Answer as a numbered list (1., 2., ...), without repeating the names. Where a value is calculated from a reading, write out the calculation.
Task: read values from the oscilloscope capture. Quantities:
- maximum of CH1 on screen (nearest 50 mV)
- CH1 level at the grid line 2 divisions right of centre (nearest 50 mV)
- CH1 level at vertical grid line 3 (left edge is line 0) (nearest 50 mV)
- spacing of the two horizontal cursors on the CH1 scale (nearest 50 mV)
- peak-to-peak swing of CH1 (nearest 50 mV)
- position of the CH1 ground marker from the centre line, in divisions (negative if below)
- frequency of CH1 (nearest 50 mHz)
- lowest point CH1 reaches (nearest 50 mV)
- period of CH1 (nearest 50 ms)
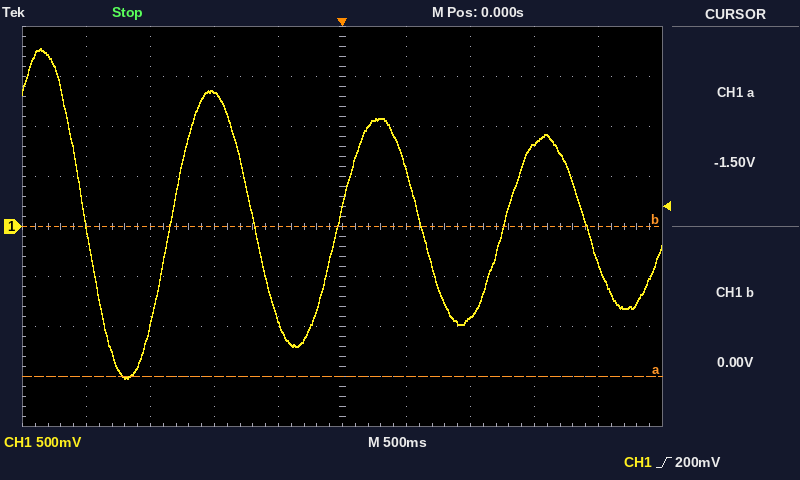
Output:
1. 1.80 V
2. -900 mV
3. 1.35 V
4. 1.50 V
5. 1.80 V − (-1.50 V) = 3.30 V
6. 0.0 div
7. 1 / 1.30 s ≈ 769 mHz, so 750 mHz to the nearest 50 mHz
8. -1.50 V
9. 1.30 s
